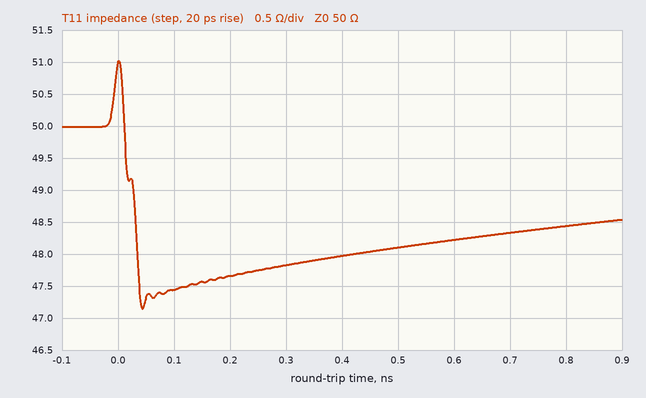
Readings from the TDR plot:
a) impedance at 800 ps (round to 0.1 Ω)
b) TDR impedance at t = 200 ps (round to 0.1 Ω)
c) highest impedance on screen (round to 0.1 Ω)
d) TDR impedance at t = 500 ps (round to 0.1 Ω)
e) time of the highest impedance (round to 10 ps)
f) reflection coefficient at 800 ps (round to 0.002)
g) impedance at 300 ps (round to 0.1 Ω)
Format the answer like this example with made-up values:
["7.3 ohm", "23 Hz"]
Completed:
["48.4 Ω", "47.7 Ω", "51.0 Ω", "48.1 Ω", "0 ps", "-0.016", "47.8 Ω"]
